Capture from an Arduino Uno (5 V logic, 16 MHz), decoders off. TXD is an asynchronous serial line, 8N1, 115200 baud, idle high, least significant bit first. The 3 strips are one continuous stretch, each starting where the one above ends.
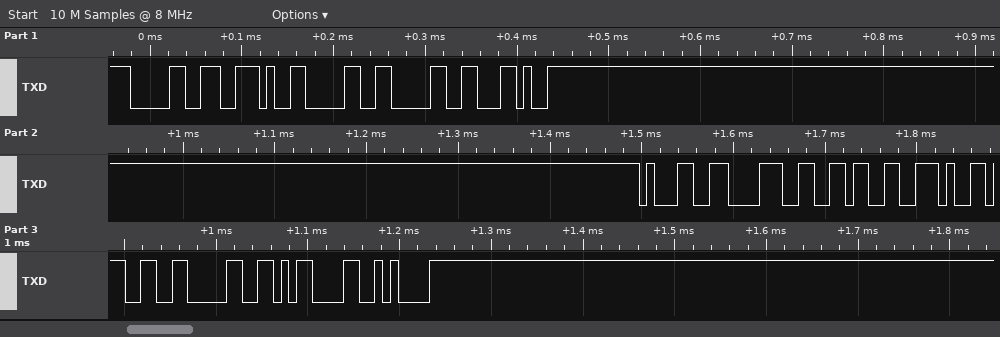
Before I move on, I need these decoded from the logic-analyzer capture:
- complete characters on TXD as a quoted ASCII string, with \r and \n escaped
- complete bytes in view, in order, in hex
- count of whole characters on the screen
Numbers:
"0.00,186.30\r\n"
30 2E 30 30 2C 31 38 36 2E 33 30 0D 0A
13
